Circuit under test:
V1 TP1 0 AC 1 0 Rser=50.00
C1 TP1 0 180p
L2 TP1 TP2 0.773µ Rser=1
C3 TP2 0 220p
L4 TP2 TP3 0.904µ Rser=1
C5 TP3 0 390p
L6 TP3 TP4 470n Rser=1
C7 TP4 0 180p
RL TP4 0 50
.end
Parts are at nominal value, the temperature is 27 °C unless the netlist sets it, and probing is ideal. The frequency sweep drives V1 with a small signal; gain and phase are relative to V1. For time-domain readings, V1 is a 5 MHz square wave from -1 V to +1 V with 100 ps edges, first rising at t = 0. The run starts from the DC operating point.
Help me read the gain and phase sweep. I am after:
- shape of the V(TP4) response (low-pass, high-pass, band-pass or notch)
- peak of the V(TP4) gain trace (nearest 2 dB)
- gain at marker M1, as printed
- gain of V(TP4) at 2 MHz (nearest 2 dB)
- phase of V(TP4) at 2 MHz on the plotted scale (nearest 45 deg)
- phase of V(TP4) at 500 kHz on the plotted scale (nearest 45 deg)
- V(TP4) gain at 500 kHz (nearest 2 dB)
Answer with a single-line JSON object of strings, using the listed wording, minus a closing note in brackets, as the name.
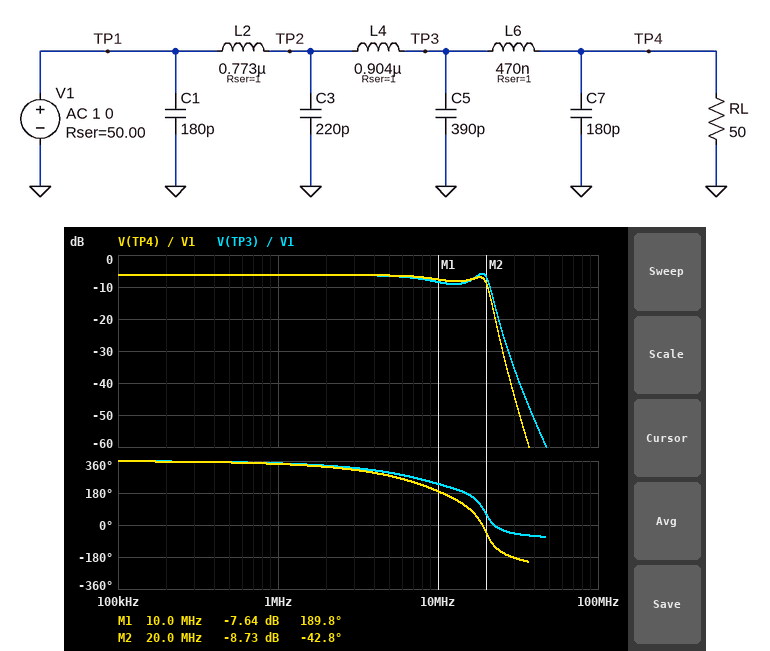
{"shape of the V(TP4) response": "low-pass", "peak of the V(TP4) gain trace": "-6 dB", "gain at marker M1, as printed": "-7.64 dB", "gain of V(TP4) at 2 MHz": "-6 dB", "phase of V(TP4) at 2 MHz on the plotted scale": "315 deg", "phase of V(TP4) at 500 kHz on the plotted scale": "360 deg", "V(TP4) gain at 500 kHz": "-6 dB"}
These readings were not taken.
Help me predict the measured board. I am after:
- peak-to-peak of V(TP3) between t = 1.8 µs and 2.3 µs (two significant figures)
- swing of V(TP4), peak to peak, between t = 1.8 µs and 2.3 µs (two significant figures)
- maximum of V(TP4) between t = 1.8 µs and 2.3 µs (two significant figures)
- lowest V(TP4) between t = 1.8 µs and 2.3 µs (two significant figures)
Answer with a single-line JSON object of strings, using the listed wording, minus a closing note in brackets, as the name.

{"peak-to-peak of V(TP3) between t = 1.8 µs and 2.3 µs": "1.1 V", "swing of V(TP4), peak to peak, between t = 1.8 µs and 2.3 µs": "1.1 V", "maximum of V(TP4) between t = 1.8 µs and 2.3 µs": "570 mV", "lowest V(TP4) between t = 1.8 µs and 2.3 µs": "-570 mV"}
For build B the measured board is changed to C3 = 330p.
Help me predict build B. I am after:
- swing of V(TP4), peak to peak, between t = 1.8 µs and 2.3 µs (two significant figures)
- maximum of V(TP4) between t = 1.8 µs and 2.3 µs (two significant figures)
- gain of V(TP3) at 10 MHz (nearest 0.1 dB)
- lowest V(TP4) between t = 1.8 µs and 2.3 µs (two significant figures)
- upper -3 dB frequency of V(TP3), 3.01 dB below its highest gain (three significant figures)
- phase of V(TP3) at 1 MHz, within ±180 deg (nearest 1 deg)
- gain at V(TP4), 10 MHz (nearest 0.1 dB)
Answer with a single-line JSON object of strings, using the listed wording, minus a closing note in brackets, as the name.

{"swing of V(TP4), peak to peak, between t = 1.8 µs and 2.3 µs": "1.3 V", "maximum of V(TP4) between t = 1.8 µs and 2.3 µs": "630 mV", "gain of V(TP3) at 10 MHz": "-7.7 dB", "lowest V(TP4) between t = 1.8 µs and 2.3 µs": "-630 mV", "upper -3 dB frequency of V(TP3), 3.01 dB below its highest gain": "17.3 MHz", "phase of V(TP3) at 1 MHz, within ±180 deg": "-14 deg", "gain at V(TP4), 10 MHz": "-6.9 dB"}
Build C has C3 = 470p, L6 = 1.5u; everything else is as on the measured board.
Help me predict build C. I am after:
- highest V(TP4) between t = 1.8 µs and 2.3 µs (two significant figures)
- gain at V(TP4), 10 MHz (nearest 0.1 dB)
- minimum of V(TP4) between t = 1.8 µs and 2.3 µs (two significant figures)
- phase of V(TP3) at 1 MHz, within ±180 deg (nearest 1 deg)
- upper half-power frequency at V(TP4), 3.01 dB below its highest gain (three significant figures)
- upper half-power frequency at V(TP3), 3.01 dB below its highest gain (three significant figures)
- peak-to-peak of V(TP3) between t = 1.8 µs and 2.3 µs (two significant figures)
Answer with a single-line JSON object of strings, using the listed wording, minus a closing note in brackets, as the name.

{"highest V(TP4) between t = 1.8 µs and 2.3 µs": "630 mV", "gain at V(TP4), 10 MHz": "-7.8 dB", "minimum of V(TP4) between t = 1.8 µs and 2.3 µs": "-630 mV", "phase of V(TP3) at 1 MHz, within ±180 deg": "-12 deg", "upper half-power frequency at V(TP4), 3.01 dB below its highest gain": "14.0 MHz", "upper half-power frequency at V(TP3), 3.01 dB below its highest gain": "14.7 MHz", "peak-to-peak of V(TP3) between t = 1.8 µs and 2.3 µs": "1.9 V"}
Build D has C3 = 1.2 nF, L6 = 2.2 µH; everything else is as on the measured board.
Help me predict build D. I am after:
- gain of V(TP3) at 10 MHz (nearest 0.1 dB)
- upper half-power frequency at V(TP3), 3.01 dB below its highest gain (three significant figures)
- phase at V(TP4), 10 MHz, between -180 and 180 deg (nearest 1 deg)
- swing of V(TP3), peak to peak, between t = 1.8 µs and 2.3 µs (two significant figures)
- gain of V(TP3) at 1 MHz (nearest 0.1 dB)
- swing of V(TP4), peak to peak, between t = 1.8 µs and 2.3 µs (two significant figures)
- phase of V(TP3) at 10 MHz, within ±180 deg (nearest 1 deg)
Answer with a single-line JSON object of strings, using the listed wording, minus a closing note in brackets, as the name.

{"gain of V(TP3) at 10 MHz": "-2.2 dB", "upper half-power frequency at V(TP3), 3.01 dB below its highest gain": "11.7 MHz", "phase at V(TP4), 10 MHz, between -180 and 180 deg": "88 deg", "swing of V(TP3), peak to peak, between t = 1.8 µs and 2.3 µs": "1.2 V", "gain of V(TP3) at 1 MHz": "-6.0 dB", "swing of V(TP4), peak to peak, between t = 1.8 µs and 2.3 µs": "750 mV", "phase of V(TP3) at 10 MHz, within ±180 deg": "-171 deg"}
